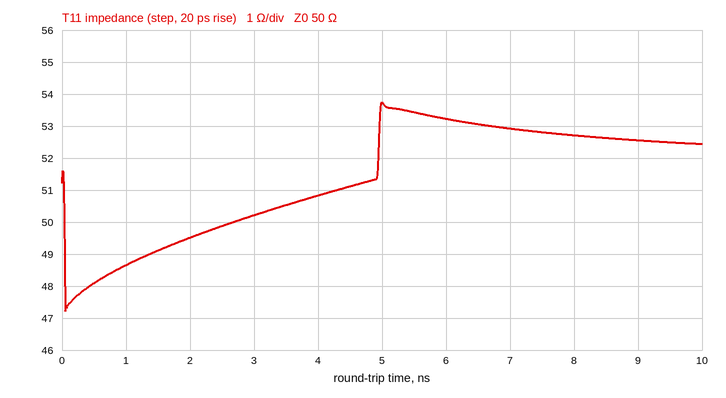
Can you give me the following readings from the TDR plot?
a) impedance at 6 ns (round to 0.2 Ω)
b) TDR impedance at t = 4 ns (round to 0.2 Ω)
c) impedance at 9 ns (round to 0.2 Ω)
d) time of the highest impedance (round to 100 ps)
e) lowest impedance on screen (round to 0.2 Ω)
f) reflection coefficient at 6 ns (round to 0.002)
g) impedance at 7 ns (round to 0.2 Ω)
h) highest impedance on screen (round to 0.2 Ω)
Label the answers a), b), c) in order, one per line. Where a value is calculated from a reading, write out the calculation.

a) 53.2 Ω
b) 50.8 Ω
c) 52.6 Ω
d) 5.0 ns
e) 47.2 Ω
f) (53.2 − 50)/(53.2 + 50) ≈ +0.0310, so +0.032 to the nearest 0.002
g) 53.0 Ω
h) 53.8 Ω
